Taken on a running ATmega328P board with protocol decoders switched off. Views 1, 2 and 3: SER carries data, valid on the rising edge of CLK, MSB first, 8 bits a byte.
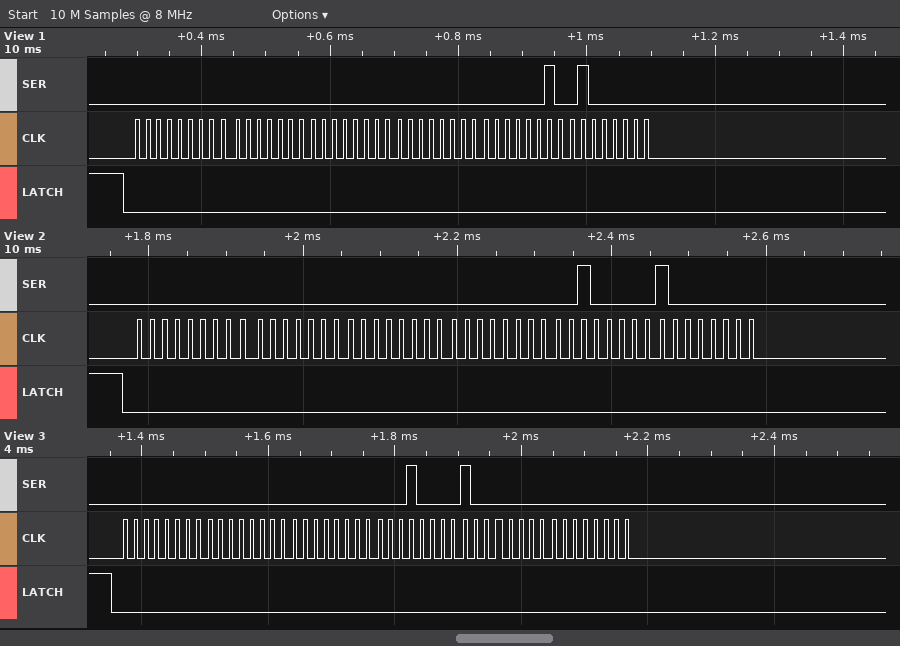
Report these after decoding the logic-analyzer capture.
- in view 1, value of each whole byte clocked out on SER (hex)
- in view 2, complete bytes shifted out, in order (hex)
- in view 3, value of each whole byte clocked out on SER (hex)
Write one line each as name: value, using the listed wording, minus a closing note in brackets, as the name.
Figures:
in view 1, value of each whole byte clocked out on SER: 00 00 00 00 02 40
in view 2, complete bytes shifted out, in order: 00 00 00 00 20 80
in view 3, value of each whole byte clocked out on SER: 0x00 0x00 0x00 0x10 0x80 0x00
